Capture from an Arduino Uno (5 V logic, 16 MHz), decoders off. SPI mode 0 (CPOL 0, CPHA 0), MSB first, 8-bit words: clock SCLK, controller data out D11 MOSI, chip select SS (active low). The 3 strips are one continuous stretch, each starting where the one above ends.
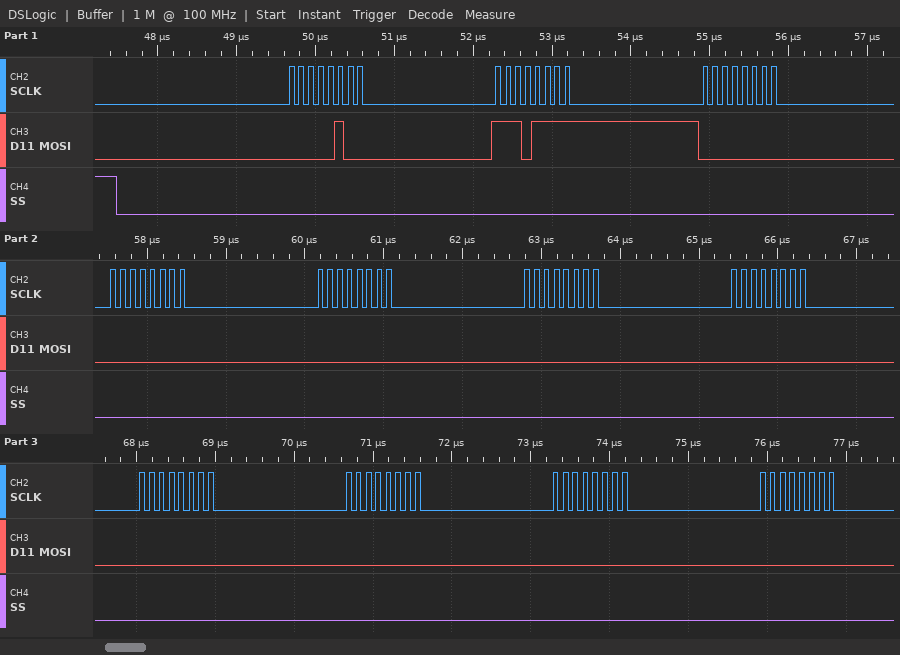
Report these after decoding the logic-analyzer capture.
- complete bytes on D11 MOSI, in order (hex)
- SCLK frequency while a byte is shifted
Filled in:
04 EF 00 00 00 00 00 00 00 00 00
8 MHz
